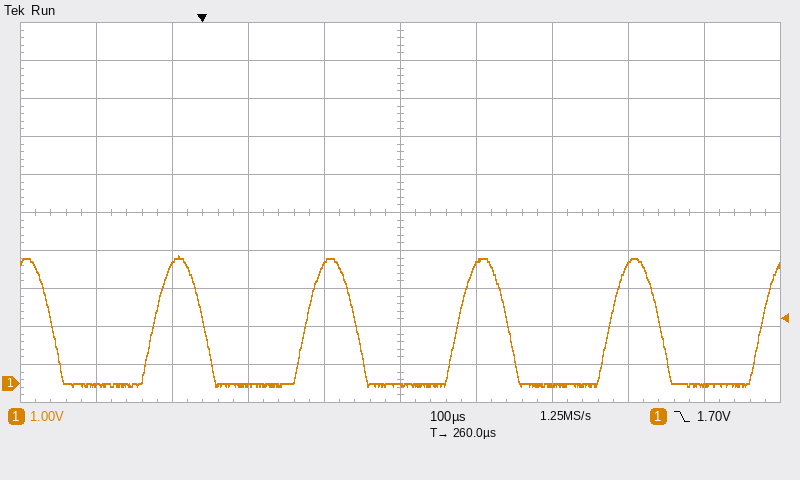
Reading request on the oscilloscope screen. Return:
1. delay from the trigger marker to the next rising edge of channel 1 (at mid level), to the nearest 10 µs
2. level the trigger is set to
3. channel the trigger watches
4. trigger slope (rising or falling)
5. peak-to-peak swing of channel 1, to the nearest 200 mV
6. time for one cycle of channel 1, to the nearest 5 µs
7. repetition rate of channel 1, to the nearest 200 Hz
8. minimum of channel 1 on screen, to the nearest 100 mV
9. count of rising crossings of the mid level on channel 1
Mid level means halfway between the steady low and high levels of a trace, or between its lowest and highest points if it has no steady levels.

140 µs
1.70 V
channel 1
falling
3.4 V
200 µs
5.0 kHz
-100 mV
5
